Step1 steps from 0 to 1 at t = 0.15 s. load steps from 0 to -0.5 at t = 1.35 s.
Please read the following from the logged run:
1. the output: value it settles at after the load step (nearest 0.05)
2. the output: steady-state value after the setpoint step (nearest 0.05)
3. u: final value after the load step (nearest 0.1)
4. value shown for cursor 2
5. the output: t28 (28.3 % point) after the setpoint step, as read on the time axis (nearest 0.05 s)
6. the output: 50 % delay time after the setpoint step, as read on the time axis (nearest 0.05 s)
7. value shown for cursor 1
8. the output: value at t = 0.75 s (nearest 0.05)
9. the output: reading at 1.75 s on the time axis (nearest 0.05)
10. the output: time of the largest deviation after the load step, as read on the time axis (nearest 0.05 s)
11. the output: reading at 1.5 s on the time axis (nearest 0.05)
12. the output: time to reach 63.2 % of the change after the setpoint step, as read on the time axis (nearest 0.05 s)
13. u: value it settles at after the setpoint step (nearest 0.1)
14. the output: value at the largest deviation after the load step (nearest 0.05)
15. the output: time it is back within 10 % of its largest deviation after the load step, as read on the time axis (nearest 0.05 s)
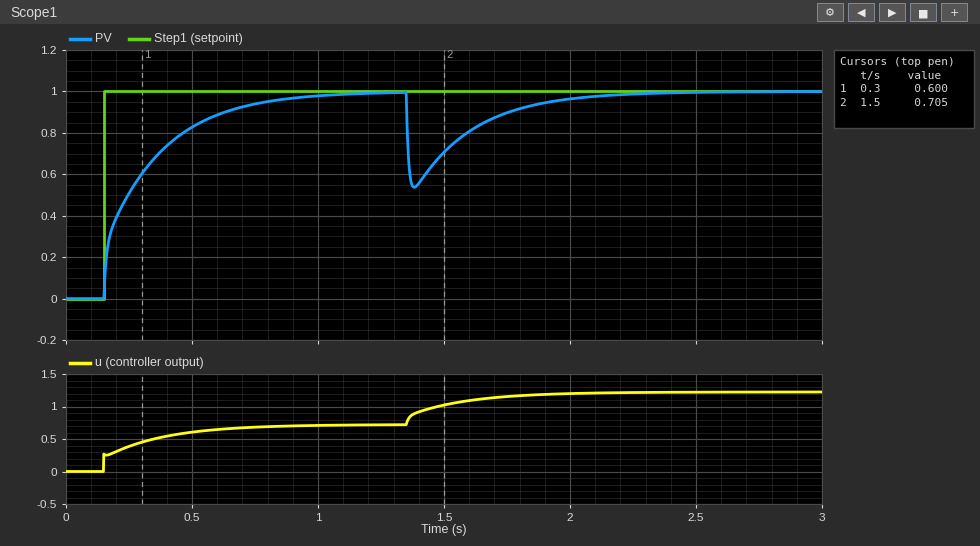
1.00
1.00
1.2
0.705
0.15 s
0.25 s
0.600
0.95
0.90
1.40 s
0.70
0.30 s
0.7
0.55
1.95 s
